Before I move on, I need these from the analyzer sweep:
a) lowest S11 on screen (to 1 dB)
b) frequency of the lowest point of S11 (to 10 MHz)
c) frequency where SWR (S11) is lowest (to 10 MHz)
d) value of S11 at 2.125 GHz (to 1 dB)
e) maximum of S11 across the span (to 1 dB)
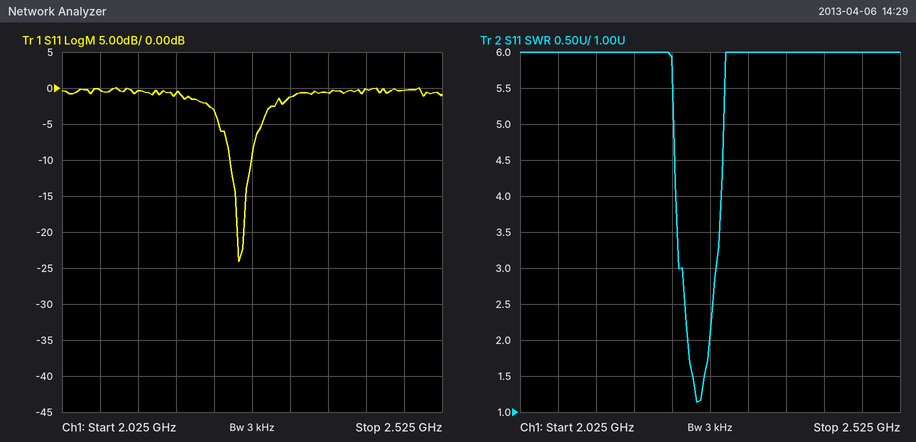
-24 dB
2.26 GHz
2.26 GHz
0 dB
0 dB
